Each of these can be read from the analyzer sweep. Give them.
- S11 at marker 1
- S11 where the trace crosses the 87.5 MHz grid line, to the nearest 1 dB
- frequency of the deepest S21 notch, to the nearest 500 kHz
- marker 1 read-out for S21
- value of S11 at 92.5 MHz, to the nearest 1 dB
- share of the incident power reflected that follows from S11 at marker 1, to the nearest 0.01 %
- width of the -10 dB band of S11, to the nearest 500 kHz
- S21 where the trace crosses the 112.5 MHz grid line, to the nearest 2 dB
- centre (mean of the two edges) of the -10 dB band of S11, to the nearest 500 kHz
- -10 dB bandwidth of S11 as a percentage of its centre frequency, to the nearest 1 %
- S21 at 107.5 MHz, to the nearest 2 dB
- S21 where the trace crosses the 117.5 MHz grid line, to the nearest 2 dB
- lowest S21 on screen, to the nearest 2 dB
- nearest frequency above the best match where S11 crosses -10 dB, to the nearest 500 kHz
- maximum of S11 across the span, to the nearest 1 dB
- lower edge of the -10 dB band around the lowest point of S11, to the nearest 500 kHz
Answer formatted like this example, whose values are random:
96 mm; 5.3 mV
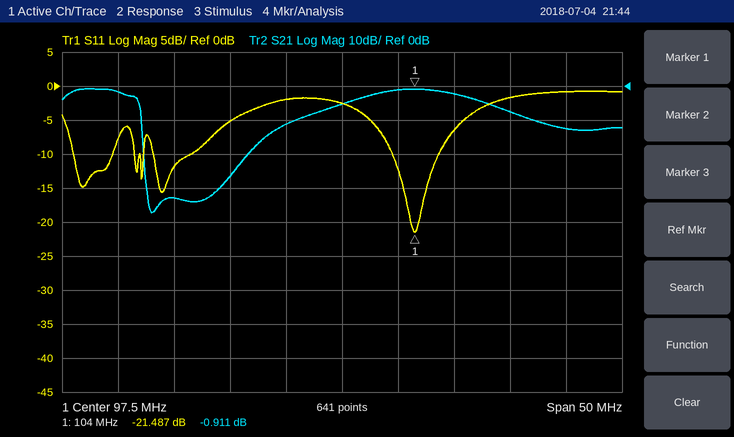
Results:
-21.487 dB; -5 dB; 80.5 MHz; -0.911 dB; -2 dB; 0.71 %; 4.0 MHz; -8 dB; 104.0 MHz; 4 %; -2 dB; -12 dB; -38 dB; 106.0 MHz; -1 dB; 102.0 MHz
